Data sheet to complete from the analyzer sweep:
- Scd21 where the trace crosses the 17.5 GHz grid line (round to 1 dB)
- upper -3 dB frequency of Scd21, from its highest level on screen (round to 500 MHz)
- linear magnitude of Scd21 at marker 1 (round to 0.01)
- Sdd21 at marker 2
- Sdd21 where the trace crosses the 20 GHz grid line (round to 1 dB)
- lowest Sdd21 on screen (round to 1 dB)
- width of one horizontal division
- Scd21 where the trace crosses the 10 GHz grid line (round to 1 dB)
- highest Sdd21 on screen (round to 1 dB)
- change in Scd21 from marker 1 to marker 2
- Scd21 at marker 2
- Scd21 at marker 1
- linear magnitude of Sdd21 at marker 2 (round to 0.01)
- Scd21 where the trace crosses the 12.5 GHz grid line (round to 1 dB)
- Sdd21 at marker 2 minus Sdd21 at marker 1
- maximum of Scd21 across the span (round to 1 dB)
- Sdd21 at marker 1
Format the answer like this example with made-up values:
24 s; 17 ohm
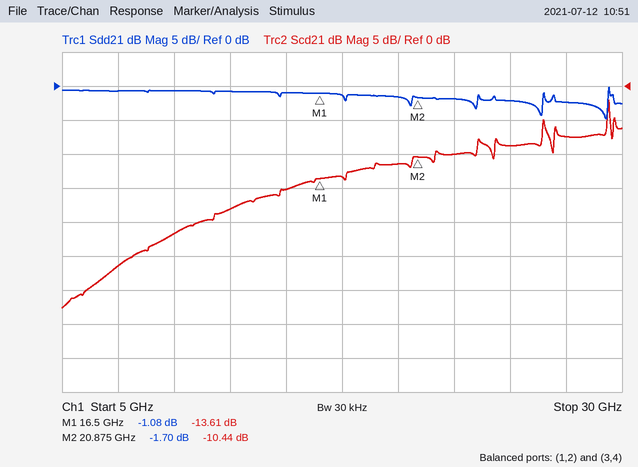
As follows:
-13 dB; 29.5 GHz; 0.21; -1.70 dB; -2 dB; -5 dB; 2.5 GHz; -22 dB; 0 dB; 3.17 dB; -10.44 dB; -13.61 dB; 0.82; -18 dB; -0.62 dB; -2 dB; -1.08 dB
